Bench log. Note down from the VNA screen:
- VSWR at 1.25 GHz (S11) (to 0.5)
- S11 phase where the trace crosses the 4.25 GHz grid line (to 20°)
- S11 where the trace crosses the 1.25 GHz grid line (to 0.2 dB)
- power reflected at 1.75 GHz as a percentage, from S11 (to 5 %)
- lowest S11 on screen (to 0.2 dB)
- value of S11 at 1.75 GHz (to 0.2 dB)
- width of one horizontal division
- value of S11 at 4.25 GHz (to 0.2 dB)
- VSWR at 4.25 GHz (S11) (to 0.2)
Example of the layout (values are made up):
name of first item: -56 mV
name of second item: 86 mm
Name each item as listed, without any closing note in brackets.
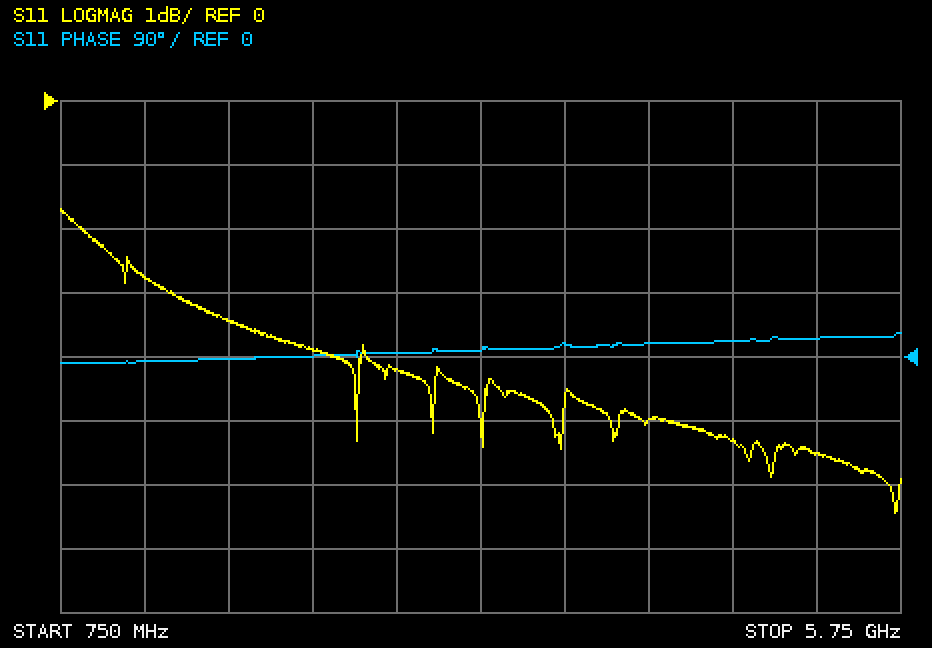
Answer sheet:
VSWR at 1.25 GHz (S11): 6.5
S11 phase where the trace crosses the 4.25 GHz grid line: 20°
S11 where the trace crosses the 1.25 GHz grid line: -2.8 dB
power reflected at 1.75 GHz as a percentage, from S11: 45 %
lowest S11 on screen: -6.4 dB
value of S11 at 1.75 GHz: -3.4 dB
width of one horizontal division: 500 MHz
value of S11 at 4.25 GHz: -5.0 dB
VSWR at 4.25 GHz (S11): 3.6
